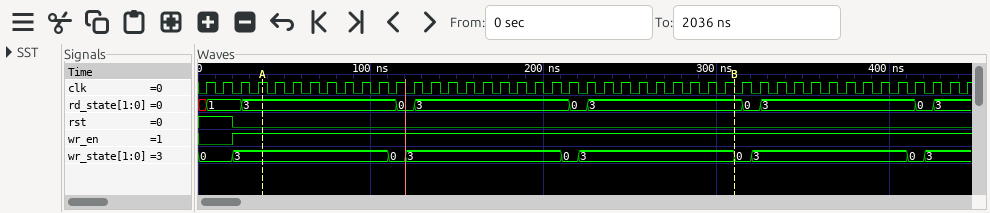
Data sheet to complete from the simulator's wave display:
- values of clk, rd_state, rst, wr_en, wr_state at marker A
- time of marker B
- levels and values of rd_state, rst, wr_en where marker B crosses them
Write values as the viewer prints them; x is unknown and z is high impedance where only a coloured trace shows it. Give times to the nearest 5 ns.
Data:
clk=1, rd_state=3, rst=0, wr_en=1, wr_state=3
310 ns
rd_state=3, rst=0, wr_en=1
